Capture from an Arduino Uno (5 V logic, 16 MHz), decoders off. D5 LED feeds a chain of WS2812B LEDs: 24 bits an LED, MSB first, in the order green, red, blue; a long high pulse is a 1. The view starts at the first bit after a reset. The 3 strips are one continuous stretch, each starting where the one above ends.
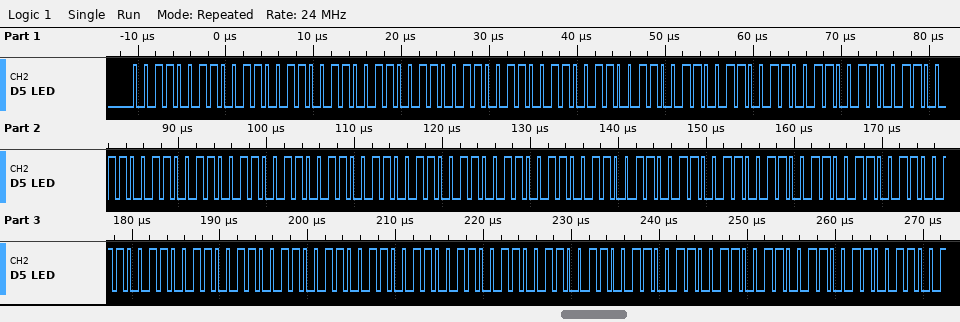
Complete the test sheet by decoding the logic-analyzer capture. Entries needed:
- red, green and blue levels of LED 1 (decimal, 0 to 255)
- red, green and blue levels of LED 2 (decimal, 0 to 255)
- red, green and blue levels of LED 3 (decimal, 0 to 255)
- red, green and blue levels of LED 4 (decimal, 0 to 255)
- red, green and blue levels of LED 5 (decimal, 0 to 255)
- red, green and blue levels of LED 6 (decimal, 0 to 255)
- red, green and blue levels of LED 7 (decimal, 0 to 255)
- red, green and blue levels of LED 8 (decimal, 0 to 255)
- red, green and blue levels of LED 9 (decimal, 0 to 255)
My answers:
51, 51, 51
51, 51, 51
51, 51, 51
51, 51, 51
51, 51, 51
51, 51, 51
51, 51, 51
51, 51, 51
51, 51, 51
